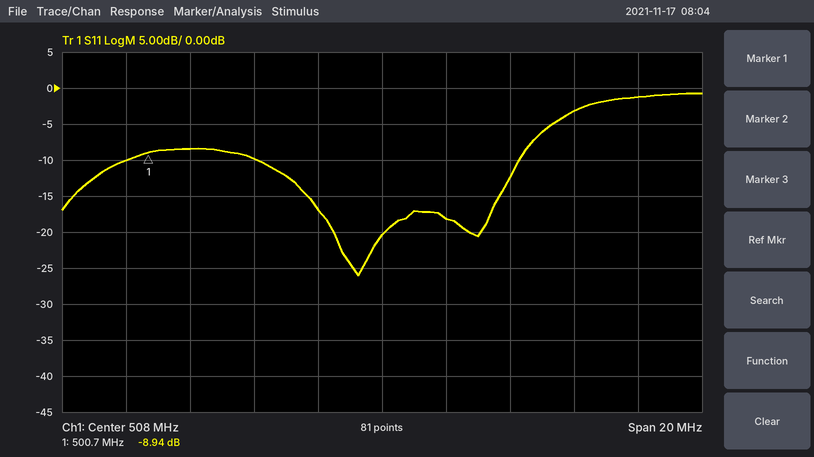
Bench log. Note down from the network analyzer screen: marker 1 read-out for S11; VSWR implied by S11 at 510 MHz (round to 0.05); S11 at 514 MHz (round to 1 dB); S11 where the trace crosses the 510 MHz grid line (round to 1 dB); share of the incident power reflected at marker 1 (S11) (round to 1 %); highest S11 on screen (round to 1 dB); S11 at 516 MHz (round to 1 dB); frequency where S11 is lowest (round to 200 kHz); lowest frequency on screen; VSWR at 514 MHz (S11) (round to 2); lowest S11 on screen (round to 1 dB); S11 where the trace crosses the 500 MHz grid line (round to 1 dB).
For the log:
-8.94 dB
1.30
-3 dB
-18 dB
13 %
-1 dB
-1 dB
507.2 MHz
498 MHz
6
-26 dB
-10 dB
